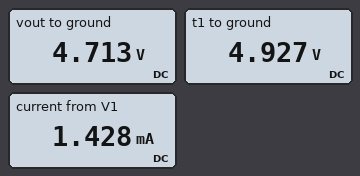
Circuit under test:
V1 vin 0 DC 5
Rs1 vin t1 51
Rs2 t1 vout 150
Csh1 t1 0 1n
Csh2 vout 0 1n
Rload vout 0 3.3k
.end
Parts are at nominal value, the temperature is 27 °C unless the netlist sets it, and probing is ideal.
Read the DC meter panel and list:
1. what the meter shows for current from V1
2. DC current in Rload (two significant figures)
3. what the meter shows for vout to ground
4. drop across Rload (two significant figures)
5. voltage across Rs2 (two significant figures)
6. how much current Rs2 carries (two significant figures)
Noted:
1.428 mA
1.4 mA
4.713 V
4.7 V
210 mV
1.4 mA
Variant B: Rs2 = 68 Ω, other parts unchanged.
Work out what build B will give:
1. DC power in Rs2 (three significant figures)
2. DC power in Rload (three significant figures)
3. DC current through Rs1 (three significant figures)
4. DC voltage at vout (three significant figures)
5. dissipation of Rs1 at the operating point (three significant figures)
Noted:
145 µW
7.06 mW
1.46 mA
4.83 V
109 µW
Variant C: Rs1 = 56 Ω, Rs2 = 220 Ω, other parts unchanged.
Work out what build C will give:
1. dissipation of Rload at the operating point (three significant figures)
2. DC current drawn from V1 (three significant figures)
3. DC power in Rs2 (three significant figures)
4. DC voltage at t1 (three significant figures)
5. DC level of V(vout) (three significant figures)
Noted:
6.45 mW
1.40 mA
430 µW
4.92 V
4.61 V
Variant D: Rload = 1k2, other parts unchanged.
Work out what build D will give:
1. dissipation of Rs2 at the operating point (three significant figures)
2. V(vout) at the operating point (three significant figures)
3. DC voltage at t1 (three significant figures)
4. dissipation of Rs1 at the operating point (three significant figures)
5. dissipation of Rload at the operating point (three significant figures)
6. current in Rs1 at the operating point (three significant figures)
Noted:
1.91 mW
4.28 V
4.82 V
650 µW
15.3 mW
3.57 mA
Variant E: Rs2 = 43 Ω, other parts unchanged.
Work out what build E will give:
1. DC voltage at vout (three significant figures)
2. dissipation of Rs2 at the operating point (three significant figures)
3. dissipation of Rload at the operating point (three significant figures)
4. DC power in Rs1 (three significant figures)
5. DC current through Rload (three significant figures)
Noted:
4.86 V
93.3 µW
7.16 mW
111 µW
1.47 mA
